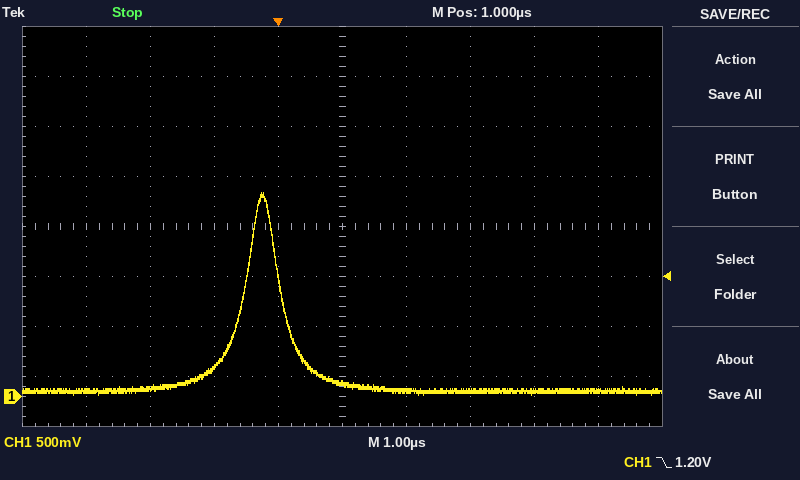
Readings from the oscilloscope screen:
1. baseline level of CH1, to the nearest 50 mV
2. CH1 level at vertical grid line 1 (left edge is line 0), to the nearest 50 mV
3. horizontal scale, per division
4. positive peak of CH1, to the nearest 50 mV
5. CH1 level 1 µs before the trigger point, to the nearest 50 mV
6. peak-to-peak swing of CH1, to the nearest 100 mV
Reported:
50 mV
50 mV
1 µs
2.05 V
300 mV
2.00 V
